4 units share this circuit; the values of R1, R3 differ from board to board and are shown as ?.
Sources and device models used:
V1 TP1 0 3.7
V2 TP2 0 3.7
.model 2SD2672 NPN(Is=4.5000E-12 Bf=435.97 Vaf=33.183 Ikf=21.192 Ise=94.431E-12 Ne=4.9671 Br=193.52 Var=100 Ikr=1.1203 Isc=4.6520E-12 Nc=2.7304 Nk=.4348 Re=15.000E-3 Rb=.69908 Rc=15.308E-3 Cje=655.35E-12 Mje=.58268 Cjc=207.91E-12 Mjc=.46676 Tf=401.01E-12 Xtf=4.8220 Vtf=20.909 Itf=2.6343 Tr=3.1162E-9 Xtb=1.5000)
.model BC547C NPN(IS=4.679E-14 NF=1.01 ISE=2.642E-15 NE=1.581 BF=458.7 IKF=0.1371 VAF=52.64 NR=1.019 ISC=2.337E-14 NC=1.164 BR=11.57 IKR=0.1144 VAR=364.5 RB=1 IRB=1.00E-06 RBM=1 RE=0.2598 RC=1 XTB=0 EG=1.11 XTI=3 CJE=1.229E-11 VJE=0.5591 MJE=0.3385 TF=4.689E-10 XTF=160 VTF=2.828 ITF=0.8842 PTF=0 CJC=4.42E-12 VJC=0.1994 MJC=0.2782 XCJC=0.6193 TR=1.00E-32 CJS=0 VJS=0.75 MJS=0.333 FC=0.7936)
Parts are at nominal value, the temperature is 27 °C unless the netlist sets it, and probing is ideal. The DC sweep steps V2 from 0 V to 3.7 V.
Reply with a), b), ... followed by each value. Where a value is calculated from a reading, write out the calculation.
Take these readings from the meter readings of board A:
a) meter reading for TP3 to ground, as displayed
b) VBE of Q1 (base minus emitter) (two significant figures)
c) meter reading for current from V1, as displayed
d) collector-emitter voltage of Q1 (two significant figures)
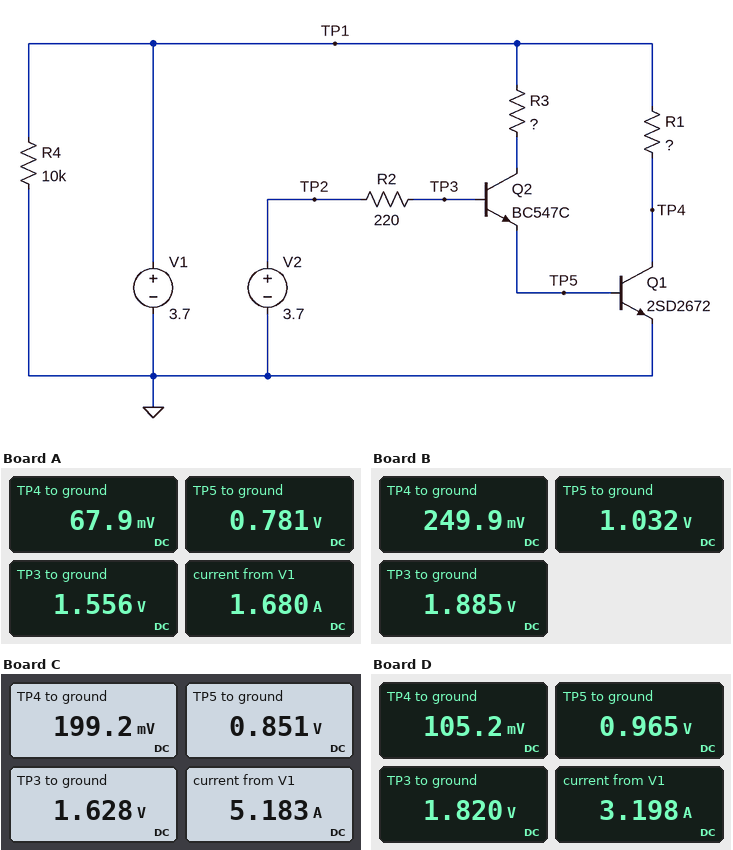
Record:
a) 1.556 V
b) 781 mV = 780 mV
c) 1.680 A
d) 67.9 mV = 68 mV
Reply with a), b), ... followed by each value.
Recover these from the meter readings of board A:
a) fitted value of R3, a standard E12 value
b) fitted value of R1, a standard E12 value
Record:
a) 100 Ω
b) 2.2 Ω
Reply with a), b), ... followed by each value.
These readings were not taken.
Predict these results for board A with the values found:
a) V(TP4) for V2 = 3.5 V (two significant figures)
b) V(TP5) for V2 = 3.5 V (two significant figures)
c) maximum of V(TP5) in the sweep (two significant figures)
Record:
a) 68 mV
b) 780 mV
c) 780 mV
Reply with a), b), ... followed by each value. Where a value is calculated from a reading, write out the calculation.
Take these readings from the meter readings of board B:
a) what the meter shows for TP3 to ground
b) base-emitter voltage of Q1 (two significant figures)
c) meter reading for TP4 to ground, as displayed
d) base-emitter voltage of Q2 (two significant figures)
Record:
a) 1.885 V
b) 1.032 V = 1.0 V
c) 249.9 mV
d) 1.885 V - 1.032 V = 850 mV
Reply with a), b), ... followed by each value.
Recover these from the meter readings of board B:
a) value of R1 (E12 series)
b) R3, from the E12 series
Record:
a) 0.47 Ω
b) 12 Ω
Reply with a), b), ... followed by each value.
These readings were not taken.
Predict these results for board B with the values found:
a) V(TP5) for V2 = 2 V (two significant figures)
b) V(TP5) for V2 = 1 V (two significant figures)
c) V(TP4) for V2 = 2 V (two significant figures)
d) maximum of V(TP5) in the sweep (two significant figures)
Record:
a) 1.0 V
b) 520 mV
c) 250 mV
d) 1.0 V
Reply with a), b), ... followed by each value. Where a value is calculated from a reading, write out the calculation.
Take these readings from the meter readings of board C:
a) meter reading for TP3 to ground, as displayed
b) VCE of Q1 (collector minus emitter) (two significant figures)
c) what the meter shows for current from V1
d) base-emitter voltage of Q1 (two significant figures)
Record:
a) 1.628 V
b) 199.2 mV = 200 mV
c) 5.183 A
d) 851 mV = 850 mV
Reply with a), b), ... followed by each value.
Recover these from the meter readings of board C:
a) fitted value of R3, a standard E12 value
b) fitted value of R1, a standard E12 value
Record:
a) 82 Ω
b) 0.68 Ω
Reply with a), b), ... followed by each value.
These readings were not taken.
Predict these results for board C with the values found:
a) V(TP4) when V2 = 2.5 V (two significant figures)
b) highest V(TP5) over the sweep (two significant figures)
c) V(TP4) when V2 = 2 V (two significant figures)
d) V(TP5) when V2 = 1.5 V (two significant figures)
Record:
a) 200 mV
b) 850 mV
c) 200 mV
d) 800 mV
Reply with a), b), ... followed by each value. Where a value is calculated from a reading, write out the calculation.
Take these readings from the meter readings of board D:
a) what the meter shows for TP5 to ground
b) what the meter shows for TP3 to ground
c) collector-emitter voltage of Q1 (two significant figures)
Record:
a) 0.965 V
b) 1.820 V
c) 105.2 mV = 110 mV
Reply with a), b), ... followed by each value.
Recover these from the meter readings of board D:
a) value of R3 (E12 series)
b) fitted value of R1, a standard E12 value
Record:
a) 12 Ω
b) 1.2 Ω
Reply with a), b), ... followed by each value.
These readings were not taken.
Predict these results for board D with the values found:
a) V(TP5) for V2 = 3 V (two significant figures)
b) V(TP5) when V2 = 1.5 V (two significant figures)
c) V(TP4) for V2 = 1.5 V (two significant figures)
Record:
a) 960 mV
b) 780 mV
c) 130 mV
